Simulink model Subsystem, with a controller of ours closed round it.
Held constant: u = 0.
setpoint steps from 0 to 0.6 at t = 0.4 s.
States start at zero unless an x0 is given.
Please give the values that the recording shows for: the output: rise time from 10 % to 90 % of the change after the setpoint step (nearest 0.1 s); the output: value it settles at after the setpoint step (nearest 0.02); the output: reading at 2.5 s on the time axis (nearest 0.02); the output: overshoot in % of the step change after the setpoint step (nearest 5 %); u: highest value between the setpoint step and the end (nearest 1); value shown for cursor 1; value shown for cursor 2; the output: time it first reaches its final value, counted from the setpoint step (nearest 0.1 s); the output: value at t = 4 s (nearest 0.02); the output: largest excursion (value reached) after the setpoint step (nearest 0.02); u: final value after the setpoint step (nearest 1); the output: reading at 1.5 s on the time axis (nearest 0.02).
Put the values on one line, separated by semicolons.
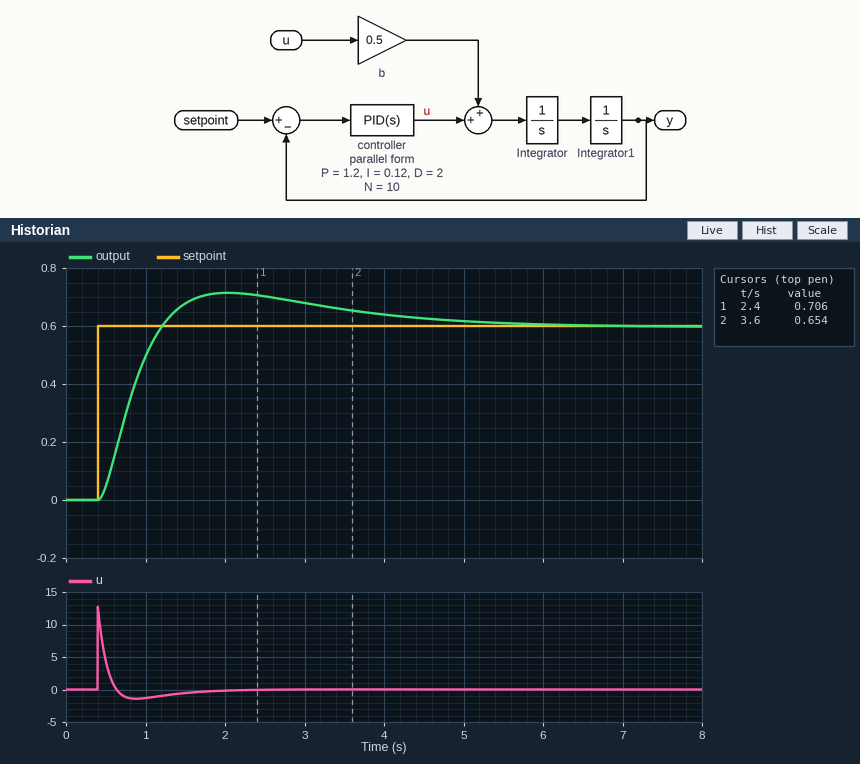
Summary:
0.6 s; 0.60; 0.70; 20 %; 13; 0.706; 0.654; 0.8 s; 0.64; 0.72; 0; 0.68
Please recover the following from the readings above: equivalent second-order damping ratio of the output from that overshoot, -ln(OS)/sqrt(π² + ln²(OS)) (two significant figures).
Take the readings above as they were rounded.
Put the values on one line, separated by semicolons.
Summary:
0.46
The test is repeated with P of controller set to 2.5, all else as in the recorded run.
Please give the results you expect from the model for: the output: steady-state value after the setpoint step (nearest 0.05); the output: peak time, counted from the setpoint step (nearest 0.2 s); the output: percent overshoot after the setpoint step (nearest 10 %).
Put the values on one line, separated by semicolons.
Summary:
0.60; 1.2 s; 30 %
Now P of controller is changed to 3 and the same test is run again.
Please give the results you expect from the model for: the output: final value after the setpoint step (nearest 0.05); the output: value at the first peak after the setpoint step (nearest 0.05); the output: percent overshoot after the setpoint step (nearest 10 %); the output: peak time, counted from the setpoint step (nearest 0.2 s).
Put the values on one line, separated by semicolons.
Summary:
0.60; 0.80; 30 %; 1.2 s
